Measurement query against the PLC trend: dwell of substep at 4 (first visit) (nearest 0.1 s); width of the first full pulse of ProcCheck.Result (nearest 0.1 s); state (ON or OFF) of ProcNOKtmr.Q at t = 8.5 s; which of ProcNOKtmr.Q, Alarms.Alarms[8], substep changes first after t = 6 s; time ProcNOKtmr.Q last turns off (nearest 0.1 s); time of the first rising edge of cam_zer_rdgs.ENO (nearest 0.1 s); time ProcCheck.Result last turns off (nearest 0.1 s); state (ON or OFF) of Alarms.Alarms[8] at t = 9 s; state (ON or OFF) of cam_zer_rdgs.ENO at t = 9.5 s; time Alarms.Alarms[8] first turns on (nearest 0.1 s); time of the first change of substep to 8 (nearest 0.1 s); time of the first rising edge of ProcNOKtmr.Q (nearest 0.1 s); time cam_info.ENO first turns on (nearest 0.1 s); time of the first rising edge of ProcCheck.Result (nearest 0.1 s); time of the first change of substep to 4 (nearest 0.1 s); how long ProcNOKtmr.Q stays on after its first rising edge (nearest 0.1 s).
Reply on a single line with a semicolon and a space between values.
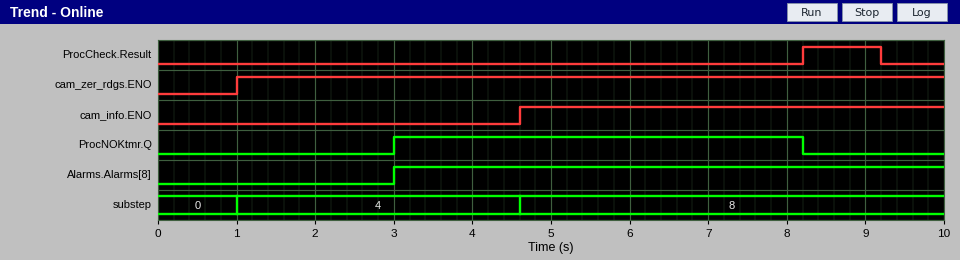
3.6 s; 1.0 s; OFF; ProcNOKtmr.Q; 8.2 s; 1.0 s; 9.2 s; ON; ON; 3.0 s; 4.6 s; 3.0 s; 4.6 s; 8.2 s; 1.0 s; 5.2 s
